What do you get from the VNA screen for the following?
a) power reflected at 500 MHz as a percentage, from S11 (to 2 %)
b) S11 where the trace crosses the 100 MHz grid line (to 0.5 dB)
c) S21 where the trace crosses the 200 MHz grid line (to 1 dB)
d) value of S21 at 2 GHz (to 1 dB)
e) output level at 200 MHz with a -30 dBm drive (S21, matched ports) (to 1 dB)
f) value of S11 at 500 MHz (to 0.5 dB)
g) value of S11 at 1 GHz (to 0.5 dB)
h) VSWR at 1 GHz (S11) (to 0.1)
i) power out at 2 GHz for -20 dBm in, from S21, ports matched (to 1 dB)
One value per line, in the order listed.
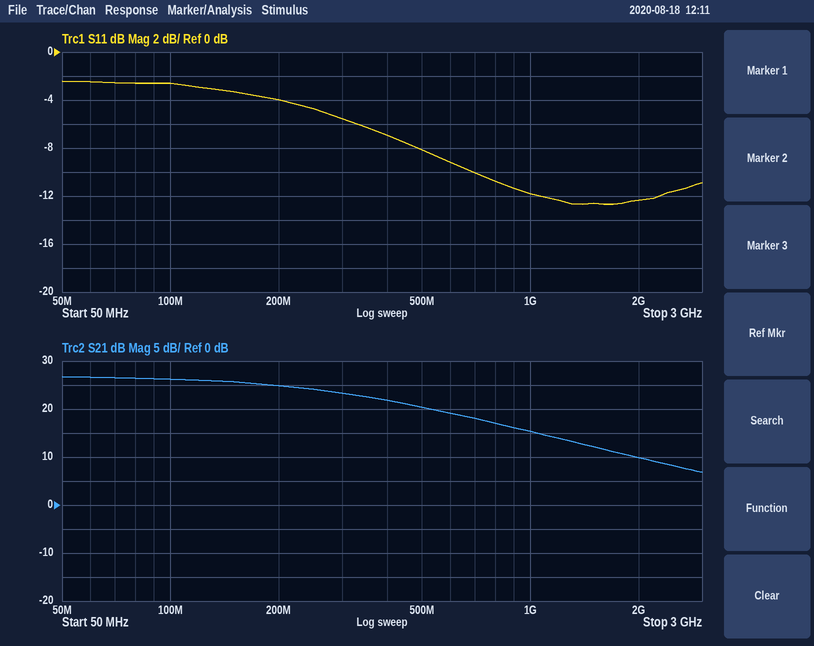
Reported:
16 %
-2.5 dB
25 dB
10 dB
-5 dBm
-8.0 dB
-12.0 dB
1.7
-10 dBm
